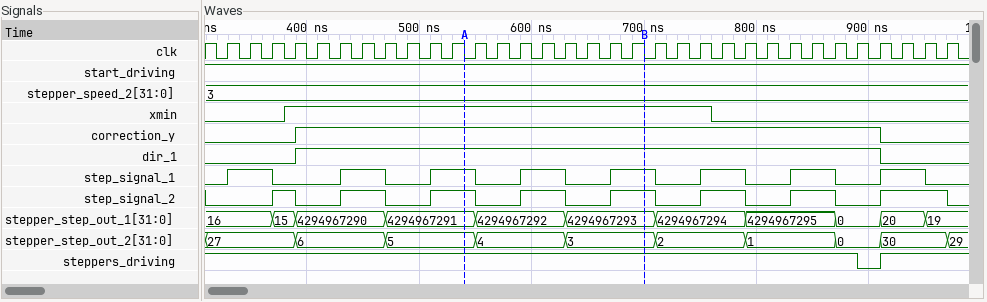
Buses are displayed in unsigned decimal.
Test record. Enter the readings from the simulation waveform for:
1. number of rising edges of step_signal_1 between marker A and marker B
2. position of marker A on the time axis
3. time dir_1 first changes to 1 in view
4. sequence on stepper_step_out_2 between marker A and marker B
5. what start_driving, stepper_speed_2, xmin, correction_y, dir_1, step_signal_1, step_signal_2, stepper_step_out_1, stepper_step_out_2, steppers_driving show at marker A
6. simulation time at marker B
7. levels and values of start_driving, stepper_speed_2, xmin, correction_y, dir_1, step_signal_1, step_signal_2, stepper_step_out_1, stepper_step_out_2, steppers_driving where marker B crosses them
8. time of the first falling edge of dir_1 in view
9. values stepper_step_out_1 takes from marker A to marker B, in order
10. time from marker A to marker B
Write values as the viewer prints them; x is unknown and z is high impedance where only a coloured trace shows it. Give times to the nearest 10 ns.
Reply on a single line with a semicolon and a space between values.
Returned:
2; 540 ns; 390 ns; 5, 4, 3; start_driving=1, stepper_speed_2=3, xmin=1, correction_y=1, dir_1=1, step_signal_1=1, step_signal_2=1, stepper_step_out_1=4294967291, stepper_step_out_2=5, steppers_driving=1; 700 ns; start_driving=1, stepper_speed_2=3, xmin=1, correction_y=1, dir_1=1, step_signal_1=1, step_signal_2=1, stepper_step_out_1=4294967293, stepper_step_out_2=3, steppers_driving=1; 910 ns; 4294967291, 4294967292, 4294967293; 160 ns
